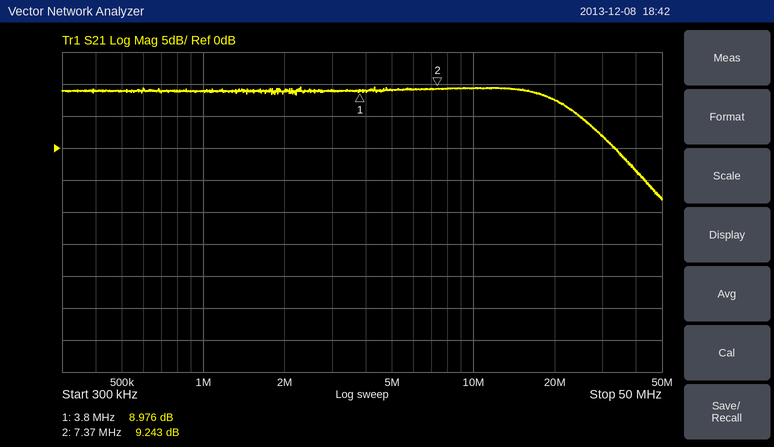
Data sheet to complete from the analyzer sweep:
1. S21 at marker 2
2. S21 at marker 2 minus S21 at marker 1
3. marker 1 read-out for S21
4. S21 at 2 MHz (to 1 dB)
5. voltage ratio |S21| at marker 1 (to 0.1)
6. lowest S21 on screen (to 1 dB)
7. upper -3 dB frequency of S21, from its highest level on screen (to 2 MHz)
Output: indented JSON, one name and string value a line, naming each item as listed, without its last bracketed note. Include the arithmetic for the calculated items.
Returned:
{
  "S21 at marker 2": "9.243 dB",
  "S21 at marker 2 minus S21 at marker 1": "9.243 − (8.976) = 0.267 dB",
  "marker 1 read-out for S21": "8.976 dB",
  "S21 at 2 MHz": "9 dB",
  "voltage ratio |S21| at marker 1": "10^(8.976/20) ≈ 2.8",
  "lowest S21 on screen": "-8 dB",
  "upper -3 dB frequency of S21, from its highest level on screen": "22 MHz"
}
